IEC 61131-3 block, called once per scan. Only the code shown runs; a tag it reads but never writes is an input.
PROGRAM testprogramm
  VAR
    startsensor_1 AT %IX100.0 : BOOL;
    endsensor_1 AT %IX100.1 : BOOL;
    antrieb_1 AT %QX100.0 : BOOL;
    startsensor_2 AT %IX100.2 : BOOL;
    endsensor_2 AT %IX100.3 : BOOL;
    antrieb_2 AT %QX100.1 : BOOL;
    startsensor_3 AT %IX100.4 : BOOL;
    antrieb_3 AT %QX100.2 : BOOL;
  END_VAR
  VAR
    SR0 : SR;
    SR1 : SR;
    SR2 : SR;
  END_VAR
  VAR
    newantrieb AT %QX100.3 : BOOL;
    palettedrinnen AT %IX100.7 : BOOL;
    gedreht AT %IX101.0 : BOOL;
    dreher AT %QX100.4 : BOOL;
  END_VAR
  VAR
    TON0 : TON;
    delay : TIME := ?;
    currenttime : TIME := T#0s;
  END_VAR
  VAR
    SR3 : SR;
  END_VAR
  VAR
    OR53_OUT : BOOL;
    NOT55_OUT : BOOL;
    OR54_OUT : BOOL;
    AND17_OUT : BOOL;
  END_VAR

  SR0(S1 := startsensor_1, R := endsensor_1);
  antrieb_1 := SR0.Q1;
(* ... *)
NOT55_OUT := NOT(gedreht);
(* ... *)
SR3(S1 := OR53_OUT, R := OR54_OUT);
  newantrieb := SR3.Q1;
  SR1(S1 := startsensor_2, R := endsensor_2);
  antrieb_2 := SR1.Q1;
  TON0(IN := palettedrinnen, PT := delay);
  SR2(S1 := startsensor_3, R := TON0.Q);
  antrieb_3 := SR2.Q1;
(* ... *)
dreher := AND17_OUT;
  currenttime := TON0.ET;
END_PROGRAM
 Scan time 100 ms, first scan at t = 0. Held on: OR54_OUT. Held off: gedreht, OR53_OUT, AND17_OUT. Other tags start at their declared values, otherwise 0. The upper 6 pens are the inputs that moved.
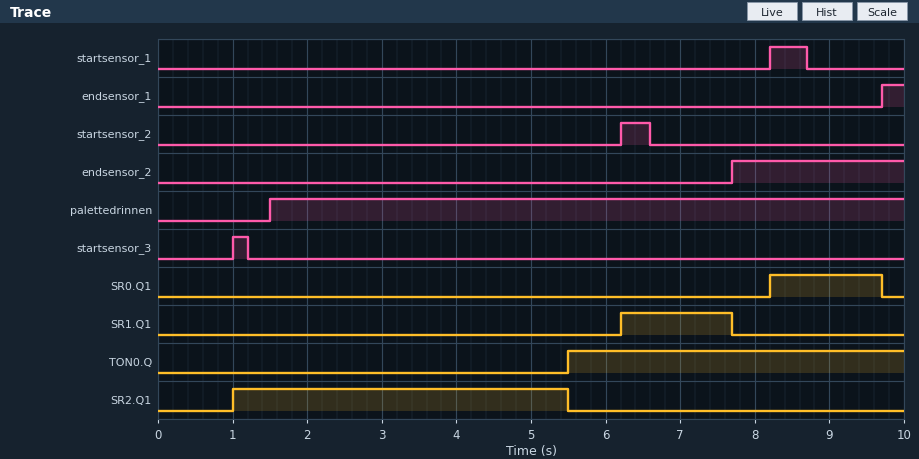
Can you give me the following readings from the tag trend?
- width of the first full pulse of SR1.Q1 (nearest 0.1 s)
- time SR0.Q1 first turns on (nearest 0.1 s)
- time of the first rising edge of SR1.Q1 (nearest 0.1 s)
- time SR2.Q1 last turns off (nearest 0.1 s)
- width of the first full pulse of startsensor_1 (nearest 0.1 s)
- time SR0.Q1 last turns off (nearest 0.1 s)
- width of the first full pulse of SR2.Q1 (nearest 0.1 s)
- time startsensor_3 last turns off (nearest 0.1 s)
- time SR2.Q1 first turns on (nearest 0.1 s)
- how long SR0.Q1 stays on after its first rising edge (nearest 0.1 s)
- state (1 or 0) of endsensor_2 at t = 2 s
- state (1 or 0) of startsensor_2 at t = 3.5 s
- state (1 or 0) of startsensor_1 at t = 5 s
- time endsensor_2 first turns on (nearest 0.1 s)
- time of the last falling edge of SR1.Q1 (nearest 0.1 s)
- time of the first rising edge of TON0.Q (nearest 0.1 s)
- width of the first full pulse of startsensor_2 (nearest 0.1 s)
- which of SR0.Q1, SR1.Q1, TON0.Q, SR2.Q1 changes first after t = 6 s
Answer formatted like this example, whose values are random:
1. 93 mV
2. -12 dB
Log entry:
1. 1.5 s
2. 8.2 s
3. 6.2 s
4. 5.5 s
5. 0.5 s
6. 9.7 s
7. 4.5 s
8. 1.2 s
9. 1.0 s
10. 1.5 s
11. 0
12. 0
13. 0
14. 7.7 s
15. 7.7 s
16. 5.5 s
17. 0.4 s
18. SR1.Q1
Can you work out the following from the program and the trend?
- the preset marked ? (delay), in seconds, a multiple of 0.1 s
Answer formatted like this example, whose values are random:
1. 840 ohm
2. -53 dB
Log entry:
1. 4.0 s
